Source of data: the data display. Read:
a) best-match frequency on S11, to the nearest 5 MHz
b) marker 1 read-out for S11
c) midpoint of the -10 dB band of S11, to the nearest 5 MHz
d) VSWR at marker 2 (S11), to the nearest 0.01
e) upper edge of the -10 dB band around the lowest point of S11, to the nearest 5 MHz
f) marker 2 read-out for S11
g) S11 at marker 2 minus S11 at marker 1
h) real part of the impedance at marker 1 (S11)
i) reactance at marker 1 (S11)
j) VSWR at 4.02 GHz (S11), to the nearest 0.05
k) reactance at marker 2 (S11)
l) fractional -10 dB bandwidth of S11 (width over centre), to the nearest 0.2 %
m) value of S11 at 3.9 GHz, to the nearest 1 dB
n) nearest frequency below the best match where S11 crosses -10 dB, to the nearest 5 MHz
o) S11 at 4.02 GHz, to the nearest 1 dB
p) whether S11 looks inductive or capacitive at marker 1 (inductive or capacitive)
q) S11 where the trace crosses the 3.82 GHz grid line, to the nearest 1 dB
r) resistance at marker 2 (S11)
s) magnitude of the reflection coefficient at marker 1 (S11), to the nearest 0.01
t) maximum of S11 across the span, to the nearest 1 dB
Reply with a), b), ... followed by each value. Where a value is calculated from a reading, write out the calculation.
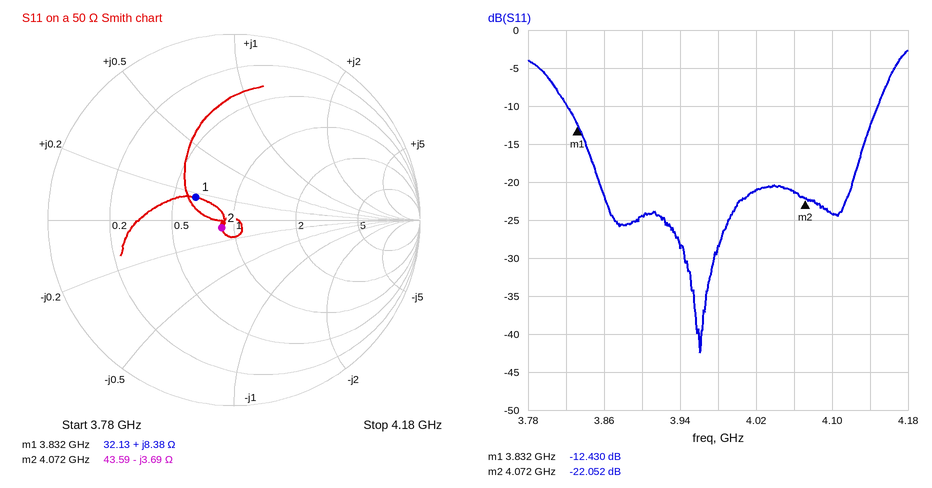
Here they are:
a) 3.960 GHz
b) -12.430 dB
c) 3.985 GHz
d) (1 + 0.0790)/(1 − 0.0790) ≈ 1.17
e) 4.150 GHz
f) -22.052 dB
g) -22.052 − (-12.43) = -9.622 dB
h) 32.13 Ω
i) +8.38 Ω
j) |Γ| = 10^(-21/20) = 0.0891; VSWR = (1 + 0.0891)/(1 − 0.0891) ≈ 1.20
k) -3.69 Ω
l) 330 MHz / 3.985 GHz ≈ 8.28 %, so 8.2 % to the nearest 0.2 %
m) -24 dB
n) 3.820 GHz
o) -21 dB
p) inductive
q) -10 dB
r) 43.59 Ω
s) 0.24
t) -3 dB
